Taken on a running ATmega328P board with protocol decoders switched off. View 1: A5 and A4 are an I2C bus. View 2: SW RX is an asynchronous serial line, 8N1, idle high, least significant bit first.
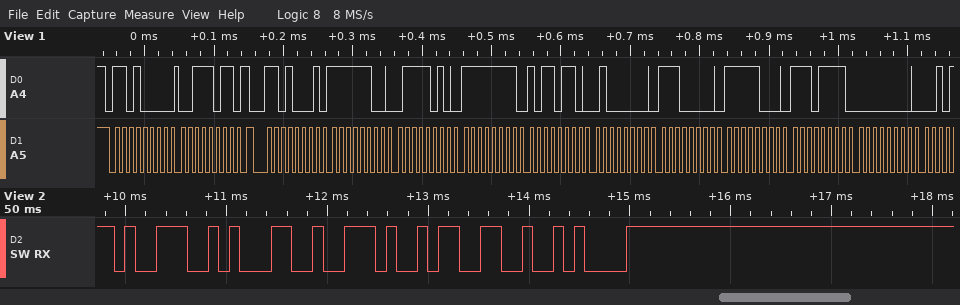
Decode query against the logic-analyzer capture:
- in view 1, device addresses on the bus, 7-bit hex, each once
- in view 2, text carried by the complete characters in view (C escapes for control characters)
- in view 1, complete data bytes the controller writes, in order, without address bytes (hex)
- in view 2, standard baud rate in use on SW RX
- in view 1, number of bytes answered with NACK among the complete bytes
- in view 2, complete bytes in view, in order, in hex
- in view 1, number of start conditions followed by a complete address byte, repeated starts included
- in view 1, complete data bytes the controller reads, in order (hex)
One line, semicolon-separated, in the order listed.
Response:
0x68; "91.3\n"; 3B; 9600 baud; 0; 39 31 2E 33 0A; 2; FC 7A FF B6 40 E0 F8 EF 00
